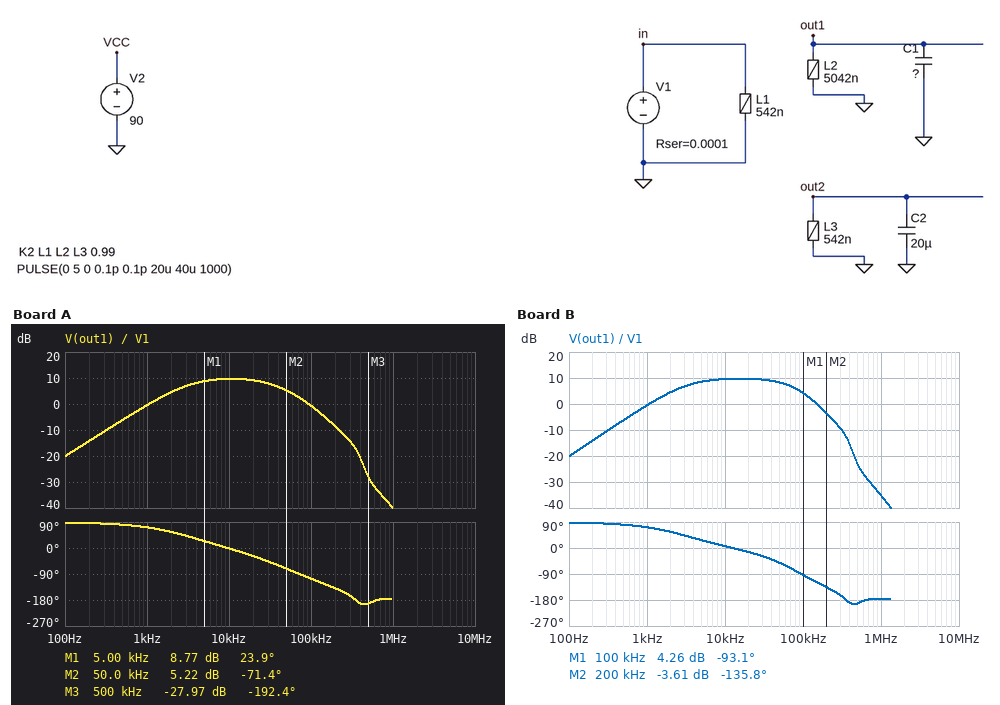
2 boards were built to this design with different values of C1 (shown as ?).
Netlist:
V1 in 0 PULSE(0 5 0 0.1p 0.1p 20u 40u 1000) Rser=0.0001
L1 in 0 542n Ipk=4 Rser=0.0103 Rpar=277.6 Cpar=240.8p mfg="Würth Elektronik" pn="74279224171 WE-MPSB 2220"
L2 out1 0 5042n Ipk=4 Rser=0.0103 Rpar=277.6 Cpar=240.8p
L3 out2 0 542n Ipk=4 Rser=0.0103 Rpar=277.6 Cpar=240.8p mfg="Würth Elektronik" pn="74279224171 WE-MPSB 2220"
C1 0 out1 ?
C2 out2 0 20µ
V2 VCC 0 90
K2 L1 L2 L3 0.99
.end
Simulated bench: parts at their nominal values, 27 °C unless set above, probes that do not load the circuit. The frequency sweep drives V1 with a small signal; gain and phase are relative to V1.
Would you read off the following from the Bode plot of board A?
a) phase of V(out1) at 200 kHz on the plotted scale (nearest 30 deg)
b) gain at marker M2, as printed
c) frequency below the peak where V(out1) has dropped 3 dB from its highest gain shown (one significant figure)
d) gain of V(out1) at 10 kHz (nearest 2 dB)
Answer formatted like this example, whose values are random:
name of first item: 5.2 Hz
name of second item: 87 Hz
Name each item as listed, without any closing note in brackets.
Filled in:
phase of V(out1) at 200 kHz on the plotted scale: -150 deg
gain at marker M2, as printed: 5.22 dB
frequency below the peak where V(out1) has dropped 3 dB from its highest gain shown: 3 kHz
gain of V(out1) at 10 kHz: 10 dB
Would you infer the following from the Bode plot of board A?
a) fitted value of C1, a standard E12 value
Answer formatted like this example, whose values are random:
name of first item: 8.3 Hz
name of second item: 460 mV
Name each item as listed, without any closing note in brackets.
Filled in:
fitted value of C1, a standard E12 value: 47 µF
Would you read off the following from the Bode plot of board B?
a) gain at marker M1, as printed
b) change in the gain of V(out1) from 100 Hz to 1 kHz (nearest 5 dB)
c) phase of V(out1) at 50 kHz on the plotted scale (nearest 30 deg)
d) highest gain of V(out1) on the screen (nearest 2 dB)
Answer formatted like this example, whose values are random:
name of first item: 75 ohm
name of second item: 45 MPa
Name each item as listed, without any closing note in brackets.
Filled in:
gain at marker M1, as printed: 4.26 dB
change in the gain of V(out1) from 100 Hz to 1 kHz: 20 dB
phase of V(out1) at 50 kHz on the plotted scale: -60 deg
highest gain of V(out1) on the screen: 10 dB
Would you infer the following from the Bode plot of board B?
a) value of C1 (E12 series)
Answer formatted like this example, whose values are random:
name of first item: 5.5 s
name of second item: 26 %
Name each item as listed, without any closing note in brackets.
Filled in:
value of C1: 27 µF
